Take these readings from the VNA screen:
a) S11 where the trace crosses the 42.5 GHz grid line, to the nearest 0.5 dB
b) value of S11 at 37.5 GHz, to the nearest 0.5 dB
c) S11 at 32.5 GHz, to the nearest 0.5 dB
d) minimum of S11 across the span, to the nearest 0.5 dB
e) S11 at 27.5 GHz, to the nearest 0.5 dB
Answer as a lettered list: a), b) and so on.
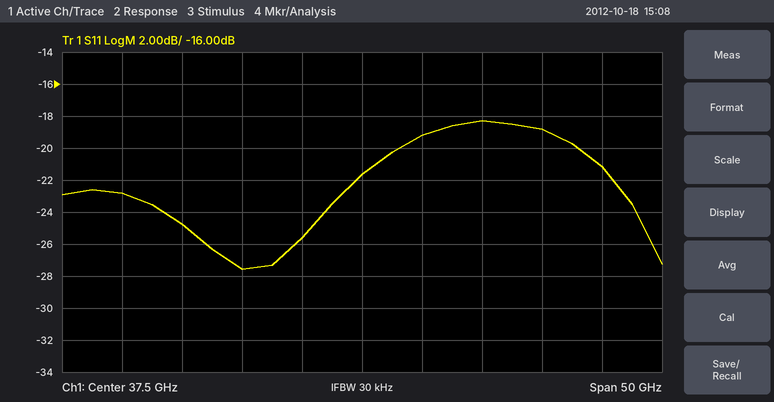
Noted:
a) -19.0 dB
b) -21.5 dB
c) -25.5 dB
d) -27.5 dB
e) -27.5 dB
